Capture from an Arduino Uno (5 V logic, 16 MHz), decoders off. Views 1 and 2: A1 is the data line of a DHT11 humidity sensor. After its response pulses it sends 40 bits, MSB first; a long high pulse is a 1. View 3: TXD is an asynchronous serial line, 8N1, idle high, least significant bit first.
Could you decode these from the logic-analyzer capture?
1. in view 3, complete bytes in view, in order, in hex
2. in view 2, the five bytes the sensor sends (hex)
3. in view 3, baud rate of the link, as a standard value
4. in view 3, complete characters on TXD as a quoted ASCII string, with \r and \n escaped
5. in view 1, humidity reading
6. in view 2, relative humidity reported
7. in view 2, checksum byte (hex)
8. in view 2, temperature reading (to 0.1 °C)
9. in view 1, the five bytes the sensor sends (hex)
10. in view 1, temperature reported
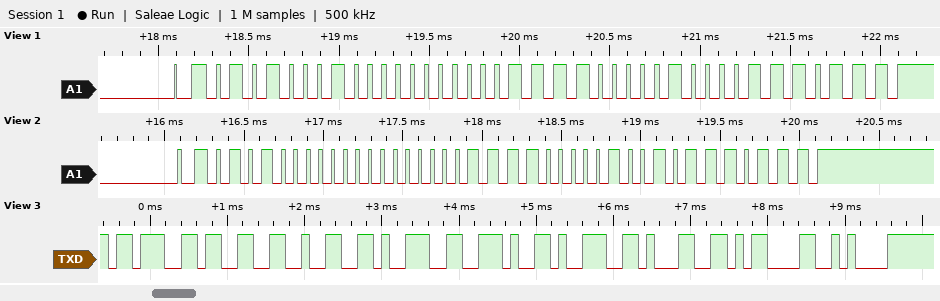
0x3B 0x33 0x32 0x39 0x2E 0x39 0x31 0x0D 0x0A
50 00 1E 09 77
9600 baud
";329.91\r\n"
81 %
80 %
0x77
30.9 °C
51 00 1E 08 77
30.8 °C
